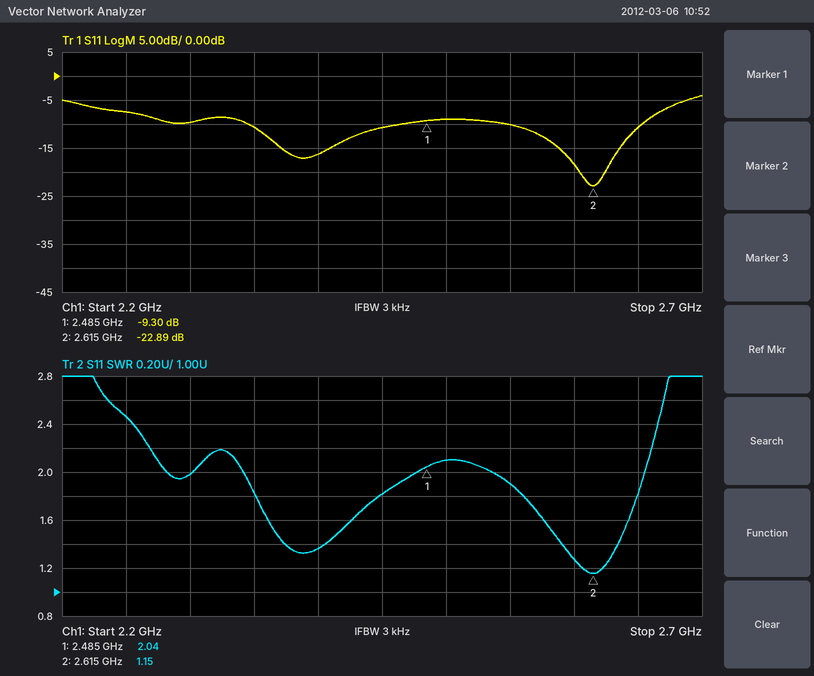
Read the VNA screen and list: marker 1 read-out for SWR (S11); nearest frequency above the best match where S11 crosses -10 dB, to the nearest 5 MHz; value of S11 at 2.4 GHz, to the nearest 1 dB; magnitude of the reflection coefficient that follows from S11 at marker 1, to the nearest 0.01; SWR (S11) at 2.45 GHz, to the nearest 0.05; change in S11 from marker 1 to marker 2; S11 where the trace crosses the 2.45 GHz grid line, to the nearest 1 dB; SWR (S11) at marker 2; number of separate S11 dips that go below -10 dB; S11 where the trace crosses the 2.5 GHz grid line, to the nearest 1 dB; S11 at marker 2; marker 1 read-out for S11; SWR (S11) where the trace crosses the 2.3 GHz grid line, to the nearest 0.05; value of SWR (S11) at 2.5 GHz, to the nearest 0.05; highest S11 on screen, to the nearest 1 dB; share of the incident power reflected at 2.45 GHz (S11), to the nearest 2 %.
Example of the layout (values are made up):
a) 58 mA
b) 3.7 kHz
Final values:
a) 2.04
b) 2.655 GHz
c) -16 dB
d) 0.34
e) 1.80
f) -13.59 dB
g) -11 dB
h) 1.15
i) 2
j) -9 dB
k) -22.89 dB
l) -9.30 dB
m) 2.00
n) 2.10
o) -4 dB
p) 8 %
